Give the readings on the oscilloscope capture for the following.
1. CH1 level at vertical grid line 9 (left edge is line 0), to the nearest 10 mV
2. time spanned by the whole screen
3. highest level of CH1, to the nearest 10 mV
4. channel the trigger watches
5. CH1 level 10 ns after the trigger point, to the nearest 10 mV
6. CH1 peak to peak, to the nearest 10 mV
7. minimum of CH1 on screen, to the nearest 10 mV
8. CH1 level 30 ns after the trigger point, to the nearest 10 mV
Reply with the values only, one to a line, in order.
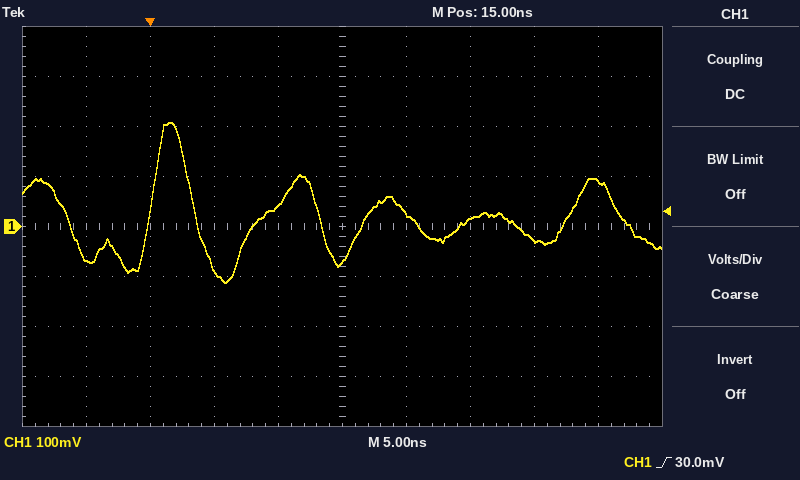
90 mV
50 ns
210 mV
CH1
40 mV
320 mV
-110 mV
-30 mV
